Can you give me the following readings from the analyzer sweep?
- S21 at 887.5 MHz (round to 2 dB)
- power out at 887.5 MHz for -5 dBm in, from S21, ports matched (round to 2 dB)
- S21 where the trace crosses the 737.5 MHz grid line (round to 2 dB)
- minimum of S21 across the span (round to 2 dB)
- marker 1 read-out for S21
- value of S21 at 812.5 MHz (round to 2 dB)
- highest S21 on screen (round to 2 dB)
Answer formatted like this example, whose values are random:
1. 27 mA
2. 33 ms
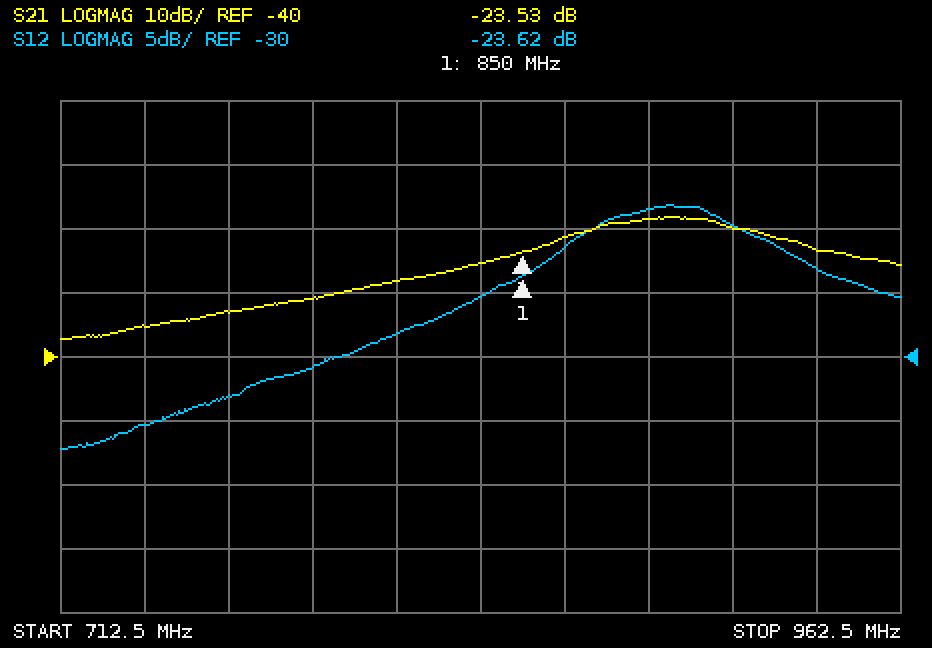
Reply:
1. -18 dB
2. -24 dBm
3. -36 dB
4. -38 dB
5. -23.53 dB
6. -28 dB
7. -18 dB
